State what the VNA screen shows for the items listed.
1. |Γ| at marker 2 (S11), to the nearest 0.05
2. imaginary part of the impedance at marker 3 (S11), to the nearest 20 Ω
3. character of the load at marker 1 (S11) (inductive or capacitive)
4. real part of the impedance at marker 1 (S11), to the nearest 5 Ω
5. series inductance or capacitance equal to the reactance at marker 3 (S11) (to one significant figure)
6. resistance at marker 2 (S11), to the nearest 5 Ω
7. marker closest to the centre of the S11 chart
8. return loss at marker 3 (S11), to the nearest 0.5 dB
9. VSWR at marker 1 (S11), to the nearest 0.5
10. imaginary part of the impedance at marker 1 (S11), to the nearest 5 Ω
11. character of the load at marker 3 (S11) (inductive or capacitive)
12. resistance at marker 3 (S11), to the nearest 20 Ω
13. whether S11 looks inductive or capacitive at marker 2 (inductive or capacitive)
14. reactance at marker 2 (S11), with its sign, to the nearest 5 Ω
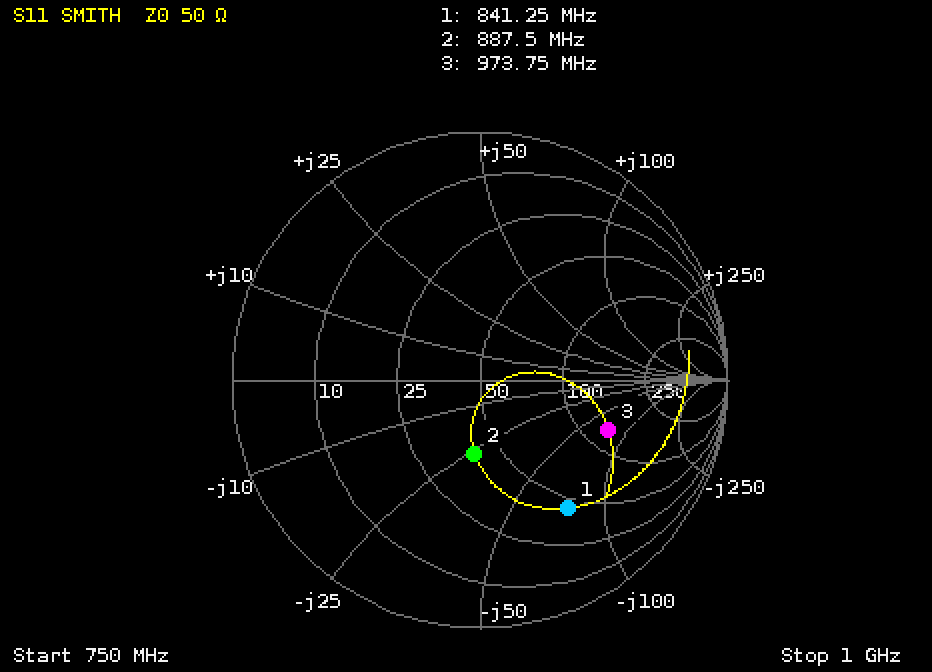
0.30
-80 Ω
capacitive
45 Ω
2 pF
40 Ω
marker 2
5.0 dB
4.5
-75 Ω
capacitive
120 Ω
capacitive
-25 Ω
